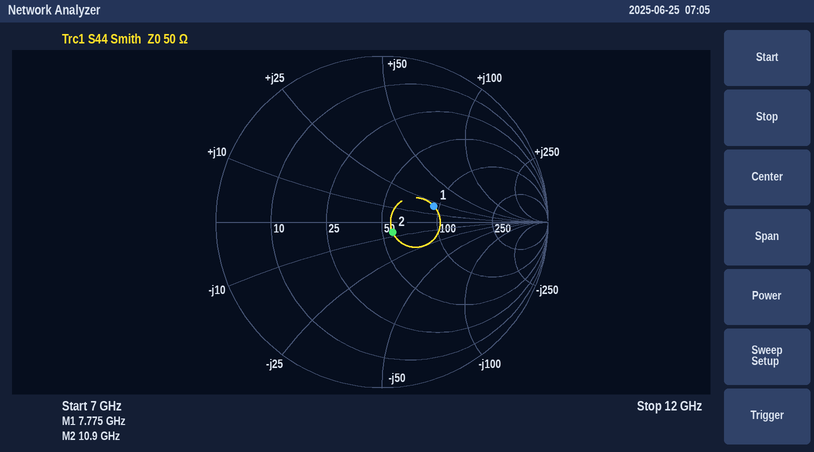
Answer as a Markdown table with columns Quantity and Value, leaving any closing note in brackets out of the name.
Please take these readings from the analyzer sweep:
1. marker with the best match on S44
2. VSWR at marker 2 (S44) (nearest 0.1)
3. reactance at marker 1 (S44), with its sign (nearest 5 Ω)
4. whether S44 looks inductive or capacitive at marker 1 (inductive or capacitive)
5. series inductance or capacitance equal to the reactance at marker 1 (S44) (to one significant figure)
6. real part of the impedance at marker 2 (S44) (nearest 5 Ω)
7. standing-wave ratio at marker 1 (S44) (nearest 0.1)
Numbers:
| Quantity | Value |
|---|---|
| marker with the best match on S44 | marker 2 |
| VSWR at marker 2 (S44) | 1.2 |
| reactance at marker 1 (S44), with its sign | +20 Ω |
| whether S44 looks inductive or capacitive at marker 1 | inductive |
| series inductance or capacitance equal to the reactance at marker 1 (S44) | 400 pH |
| real part of the impedance at marker 2 (S44) | 55 Ω |
| standing-wave ratio at marker 1 (S44) | 2.0 |
